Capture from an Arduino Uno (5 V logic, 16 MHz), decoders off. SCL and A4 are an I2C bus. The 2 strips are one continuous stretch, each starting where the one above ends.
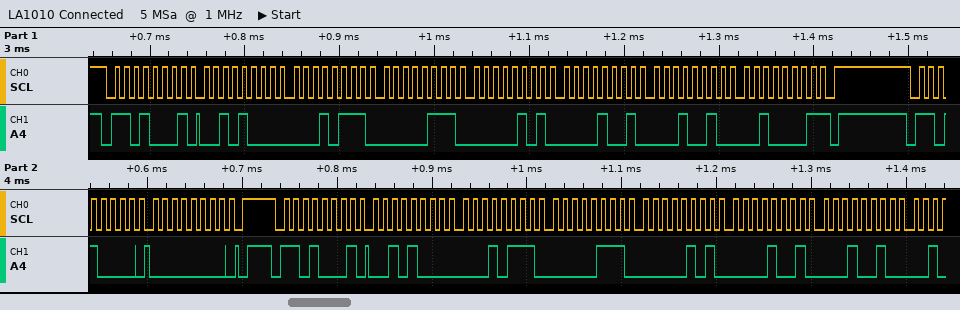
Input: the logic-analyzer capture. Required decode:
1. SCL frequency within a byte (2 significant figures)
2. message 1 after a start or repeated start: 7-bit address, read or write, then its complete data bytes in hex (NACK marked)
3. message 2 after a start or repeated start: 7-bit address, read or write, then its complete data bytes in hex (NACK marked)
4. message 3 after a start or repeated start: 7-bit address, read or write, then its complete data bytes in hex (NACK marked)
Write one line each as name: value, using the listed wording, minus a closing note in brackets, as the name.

SCL frequency within a byte: 100 kHz
message 1 after a start or repeated start: 7-bit address, read or write, then its complete data bytes in hex: 0x68 read: 28 17 07 05 09 12 21 NACK
message 2 after a start or repeated start: 7-bit address, read or write, then its complete data bytes in hex: 0x68 write: 00
message 3 after a start or repeated start: 7-bit address, read or write, then its complete data bytes in hex: 0x68 read: 28 17 07 05 09 12
